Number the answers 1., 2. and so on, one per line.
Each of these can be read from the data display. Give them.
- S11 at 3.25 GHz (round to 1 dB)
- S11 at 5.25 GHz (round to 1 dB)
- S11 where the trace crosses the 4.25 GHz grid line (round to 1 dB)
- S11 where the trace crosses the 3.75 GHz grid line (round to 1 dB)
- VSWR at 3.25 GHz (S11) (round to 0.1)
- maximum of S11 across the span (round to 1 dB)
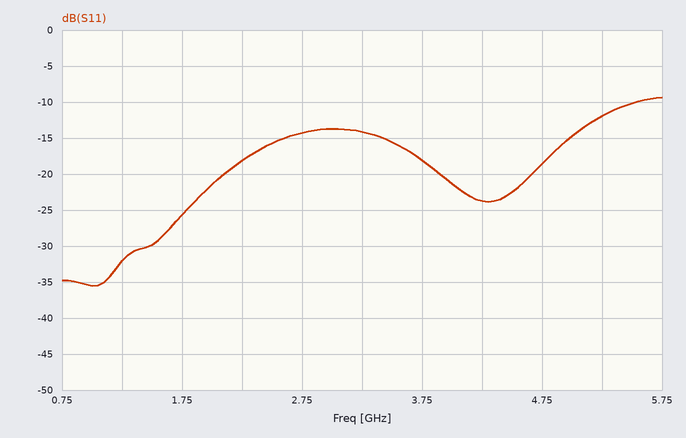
1. -14 dB
2. -12 dB
3. -24 dB
4. -18 dB
5. 1.5
6. -9 dB
